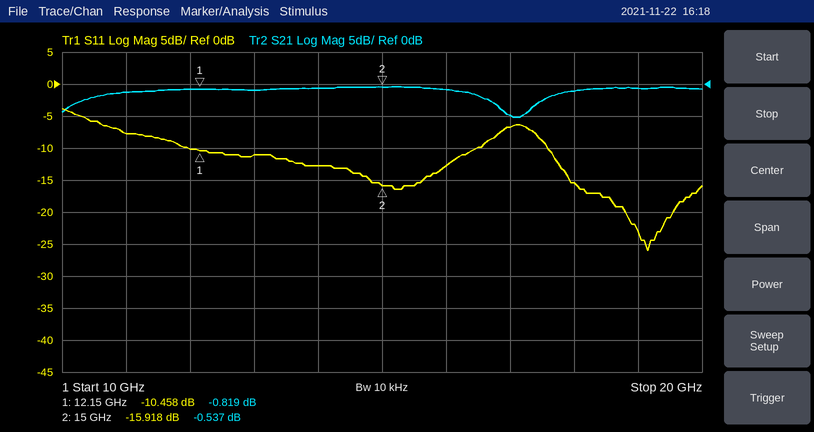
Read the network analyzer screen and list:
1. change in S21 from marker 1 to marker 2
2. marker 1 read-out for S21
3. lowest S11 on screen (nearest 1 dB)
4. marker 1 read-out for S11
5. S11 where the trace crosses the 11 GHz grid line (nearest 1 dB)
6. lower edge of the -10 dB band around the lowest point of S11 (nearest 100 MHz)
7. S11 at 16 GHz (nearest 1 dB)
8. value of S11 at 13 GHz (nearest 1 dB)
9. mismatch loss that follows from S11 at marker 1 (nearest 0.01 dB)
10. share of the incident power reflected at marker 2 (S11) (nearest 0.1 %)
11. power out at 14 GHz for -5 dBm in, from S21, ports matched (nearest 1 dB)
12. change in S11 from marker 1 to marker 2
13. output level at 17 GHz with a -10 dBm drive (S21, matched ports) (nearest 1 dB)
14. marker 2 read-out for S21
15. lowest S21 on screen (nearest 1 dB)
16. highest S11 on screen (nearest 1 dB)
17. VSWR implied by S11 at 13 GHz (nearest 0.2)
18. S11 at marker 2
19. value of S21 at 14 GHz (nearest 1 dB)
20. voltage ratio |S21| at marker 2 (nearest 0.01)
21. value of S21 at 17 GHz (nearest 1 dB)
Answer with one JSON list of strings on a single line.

["0.282 dB", "-0.819 dB", "-26 dB", "-10.458 dB", "-8 dB", "17.6 GHz", "-13 dB", "-11 dB", "0.41 dB", "2.6 %", "-6 dBm", "-5.460 dB", "-15 dBm", "-0.537 dB", "-5 dB", "-4 dB", "1.8", "-15.918 dB", "-1 dB", "0.94", "-5 dB"]
